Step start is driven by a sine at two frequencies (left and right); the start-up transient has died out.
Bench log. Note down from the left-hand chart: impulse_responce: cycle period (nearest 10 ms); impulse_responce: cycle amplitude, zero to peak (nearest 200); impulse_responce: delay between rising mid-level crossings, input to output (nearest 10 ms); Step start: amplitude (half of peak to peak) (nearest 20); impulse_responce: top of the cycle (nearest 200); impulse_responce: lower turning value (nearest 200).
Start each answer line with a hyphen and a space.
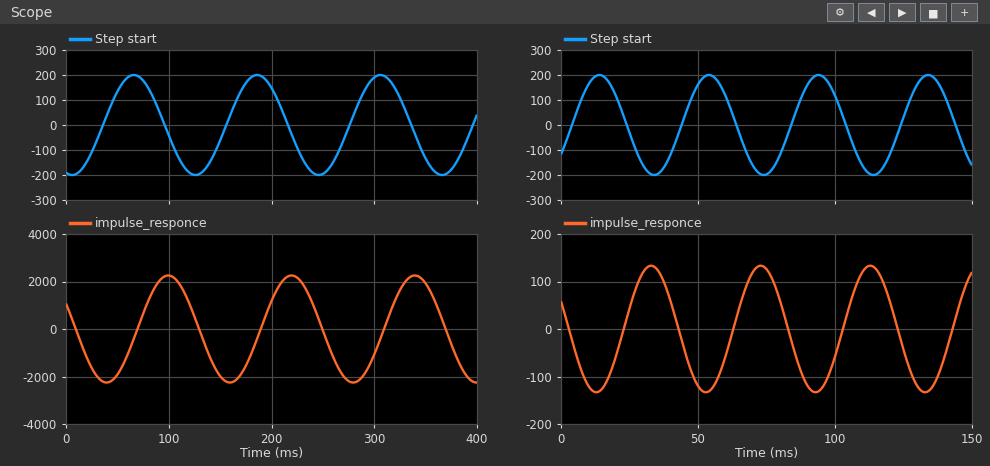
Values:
- 120 ms
- 2200
- 30 ms
- 200
- 2200
- -2200
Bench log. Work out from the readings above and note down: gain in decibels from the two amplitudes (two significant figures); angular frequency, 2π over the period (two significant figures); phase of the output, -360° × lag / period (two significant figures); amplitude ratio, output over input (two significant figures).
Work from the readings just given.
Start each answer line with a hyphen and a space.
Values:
- 21 dB
- 0.052 rad/ms
- -90°
- 11
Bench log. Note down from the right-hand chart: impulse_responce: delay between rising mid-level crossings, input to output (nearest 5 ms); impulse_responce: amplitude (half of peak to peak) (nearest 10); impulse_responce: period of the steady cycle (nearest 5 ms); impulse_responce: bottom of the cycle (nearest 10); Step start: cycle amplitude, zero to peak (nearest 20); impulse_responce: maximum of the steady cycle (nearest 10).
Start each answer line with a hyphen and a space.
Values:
- 20 ms
- 130
- 40 ms
- -130
- 200
- 130
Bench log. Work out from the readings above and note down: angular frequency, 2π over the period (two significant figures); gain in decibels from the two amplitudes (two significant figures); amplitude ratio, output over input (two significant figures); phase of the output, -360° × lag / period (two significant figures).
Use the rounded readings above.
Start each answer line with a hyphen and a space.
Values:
- 0.16 rad/ms
- -3.7 dB
- 0.65
- -180°
